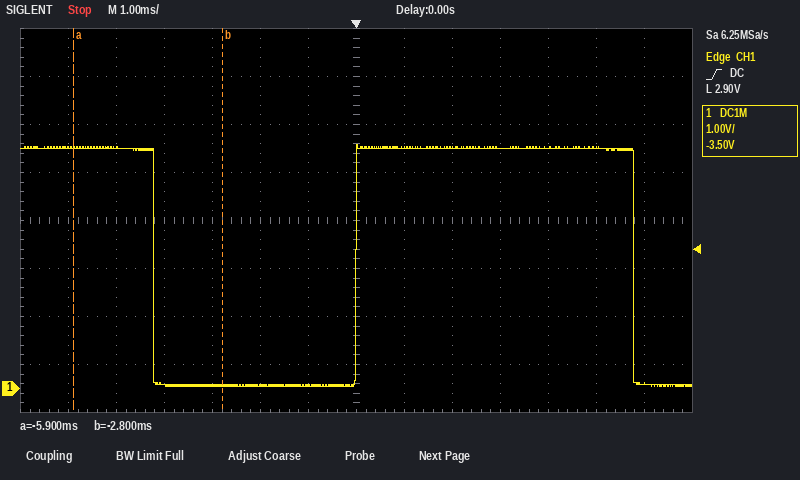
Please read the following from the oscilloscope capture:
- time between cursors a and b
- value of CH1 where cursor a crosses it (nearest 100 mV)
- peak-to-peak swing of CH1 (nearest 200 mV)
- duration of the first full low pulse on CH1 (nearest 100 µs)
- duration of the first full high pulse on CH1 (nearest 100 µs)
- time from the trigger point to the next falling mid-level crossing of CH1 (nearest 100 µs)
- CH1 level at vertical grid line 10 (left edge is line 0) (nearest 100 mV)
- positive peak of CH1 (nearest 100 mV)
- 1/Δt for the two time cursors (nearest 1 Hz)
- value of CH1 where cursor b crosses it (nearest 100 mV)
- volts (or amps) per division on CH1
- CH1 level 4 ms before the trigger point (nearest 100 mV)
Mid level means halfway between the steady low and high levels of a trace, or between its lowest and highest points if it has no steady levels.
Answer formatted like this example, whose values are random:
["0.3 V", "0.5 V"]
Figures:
["3.1 ms", "5.0 V", "5.0 V", "4.2 ms", "5.8 ms", "5.8 ms", "5.0 V", "5.1 V", "323 Hz", "100 mV", "1 V", "100 mV"]
